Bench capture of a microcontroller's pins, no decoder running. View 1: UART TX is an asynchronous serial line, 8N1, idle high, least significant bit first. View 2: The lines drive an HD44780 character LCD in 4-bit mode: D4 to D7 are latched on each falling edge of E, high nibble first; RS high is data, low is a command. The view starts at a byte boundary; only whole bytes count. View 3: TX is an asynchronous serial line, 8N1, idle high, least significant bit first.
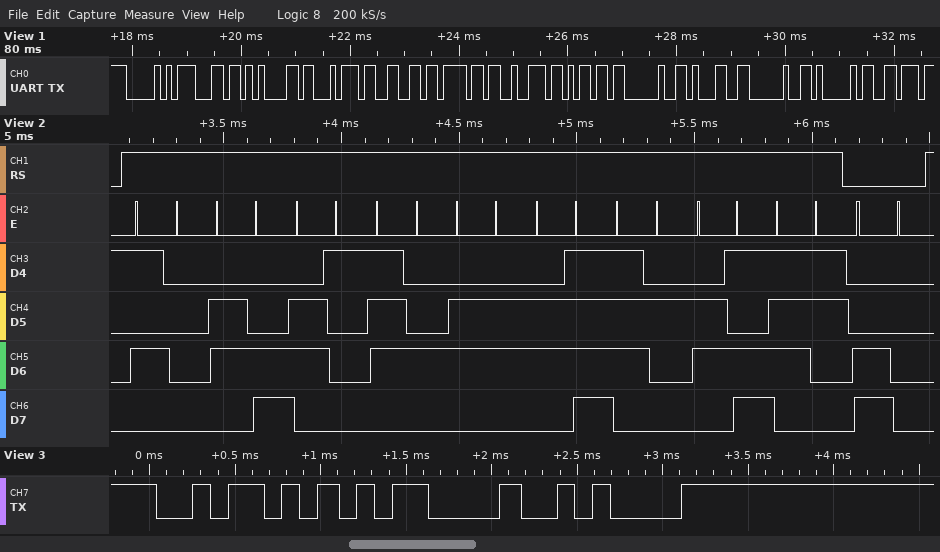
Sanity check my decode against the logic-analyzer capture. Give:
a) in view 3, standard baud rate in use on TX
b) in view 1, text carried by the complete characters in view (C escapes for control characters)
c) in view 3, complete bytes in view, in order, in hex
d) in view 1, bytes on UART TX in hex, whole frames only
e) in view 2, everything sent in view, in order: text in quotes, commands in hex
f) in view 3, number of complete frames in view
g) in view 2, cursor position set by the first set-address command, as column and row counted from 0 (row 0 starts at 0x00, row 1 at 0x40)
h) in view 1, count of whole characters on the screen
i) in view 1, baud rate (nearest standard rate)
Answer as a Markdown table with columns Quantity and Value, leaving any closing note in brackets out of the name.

| Quantity | Value |
|---|---|
| in view 3, standard baud rate in use on TX | 9600 baud |
| in view 1, text carried by the complete characters in view | "Platform 1 Av" |
| in view 3, complete bytes in view, in order, in hex | 0x5A 0x0D 0x0A |
| in view 1, bytes on UART TX in hex, whole frames only | 50 6C 61 74 66 6F 72 6D 20 31 20 41 76 |
| in view 2, everything sent in view, in order: text in quotes, commands in hex | "Platforms" 0xC0 |
| in view 3, number of complete frames in view | 3 |
| in view 2, cursor position set by the first set-address command, as column and row counted from 0 | column 0, row 1 |
| in view 1, count of whole characters on the screen | 13 |
| in view 1, baud rate | 9600 baud |
